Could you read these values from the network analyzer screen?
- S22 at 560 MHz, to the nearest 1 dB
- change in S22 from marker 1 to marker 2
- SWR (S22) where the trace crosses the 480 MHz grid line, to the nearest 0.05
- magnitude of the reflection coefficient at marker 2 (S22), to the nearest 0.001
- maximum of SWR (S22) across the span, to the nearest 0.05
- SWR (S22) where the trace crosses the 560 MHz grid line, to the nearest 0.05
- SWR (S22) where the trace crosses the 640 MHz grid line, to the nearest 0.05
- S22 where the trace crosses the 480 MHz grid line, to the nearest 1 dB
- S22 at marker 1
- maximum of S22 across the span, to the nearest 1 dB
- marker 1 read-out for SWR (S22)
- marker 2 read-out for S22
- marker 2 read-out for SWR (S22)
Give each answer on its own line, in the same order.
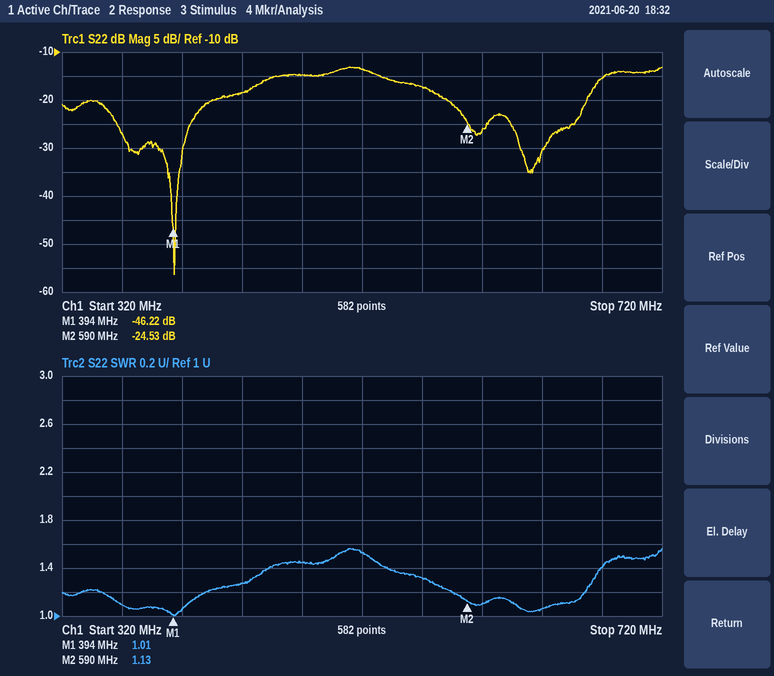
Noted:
-17 dB
21.69 dB
1.45
0.059
1.55
1.30
1.05
-15 dB
-46.22 dB
-13 dB
1.01
-24.53 dB
1.13
